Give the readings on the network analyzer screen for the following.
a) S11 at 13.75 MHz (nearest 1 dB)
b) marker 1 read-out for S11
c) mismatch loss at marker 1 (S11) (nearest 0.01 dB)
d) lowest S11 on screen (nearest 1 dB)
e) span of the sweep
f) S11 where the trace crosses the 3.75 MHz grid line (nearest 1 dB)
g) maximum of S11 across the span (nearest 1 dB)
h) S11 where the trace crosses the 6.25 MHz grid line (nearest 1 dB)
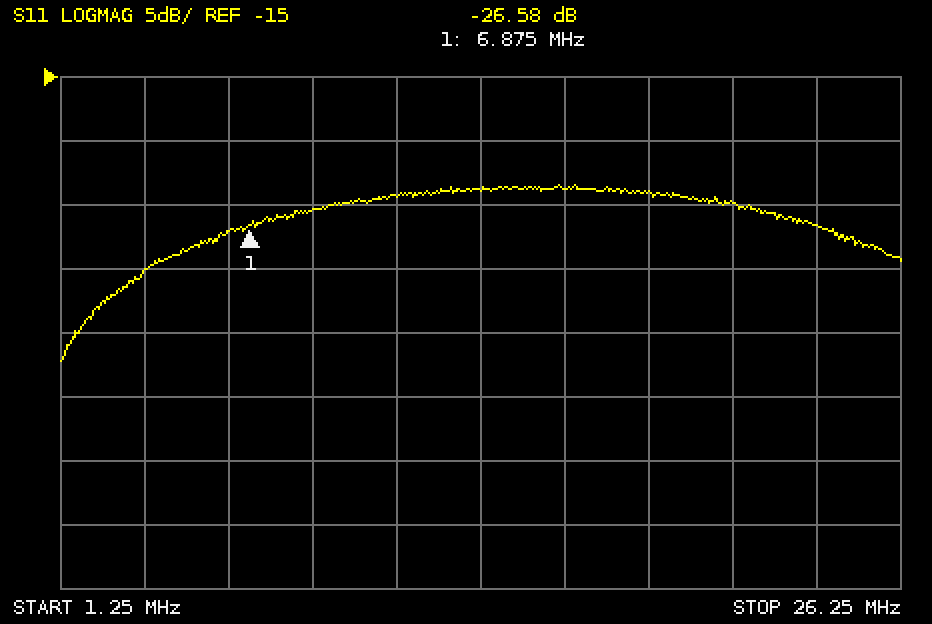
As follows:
-24 dB
-26.58 dB
0.01 dB
-37 dB
25 MHz
-30 dB
-23 dB
-27 dB
